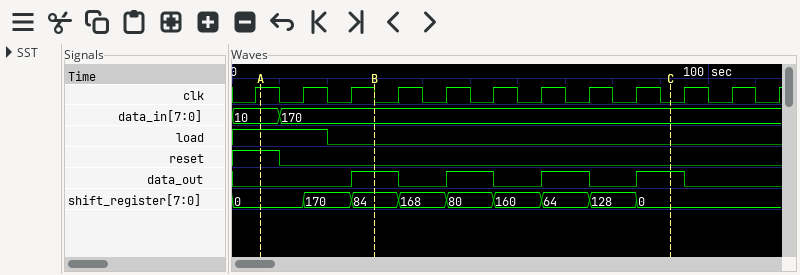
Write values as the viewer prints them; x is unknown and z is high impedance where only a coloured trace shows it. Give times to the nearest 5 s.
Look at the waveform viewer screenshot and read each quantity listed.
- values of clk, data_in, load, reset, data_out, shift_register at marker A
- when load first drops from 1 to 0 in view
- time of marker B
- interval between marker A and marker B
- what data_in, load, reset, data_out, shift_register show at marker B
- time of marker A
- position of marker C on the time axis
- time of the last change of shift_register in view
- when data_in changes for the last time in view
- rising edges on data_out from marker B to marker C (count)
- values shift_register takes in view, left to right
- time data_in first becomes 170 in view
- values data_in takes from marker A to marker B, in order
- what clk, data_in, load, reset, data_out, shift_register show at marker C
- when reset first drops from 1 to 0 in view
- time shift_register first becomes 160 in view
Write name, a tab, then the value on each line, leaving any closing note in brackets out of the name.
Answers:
values of clk, data_in, load, reset, data_out, shift_register at marker A	clk=1, data_in=10, load=1, reset=1, data_out=0, shift_register=0
when load first drops from 1 to 0 in view	20 s
time of marker B	30 s
interval between marker A and marker B	25 s
what data_in, load, reset, data_out, shift_register show at marker B	data_in=170, load=0, reset=0, data_out=1, shift_register=84
time of marker A	5 s
position of marker C on the time axis	90 s
time of the last change of shift_register in view	85 s
when data_in changes for the last time in view	10 s
rising edges on data_out from marker B to marker C	3
values shift_register takes in view, left to right	0, 170, 84, 168, 80, 160, 64, 128, 0
time data_in first becomes 170 in view	10 s
values data_in takes from marker A to marker B, in order	10, 170
what clk, data_in, load, reset, data_out, shift_register show at marker C	clk=0, data_in=170, load=0, reset=0, data_out=1, shift_register=0
when reset first drops from 1 to 0 in view	10 s
time shift_register first becomes 160 in view	55 s
